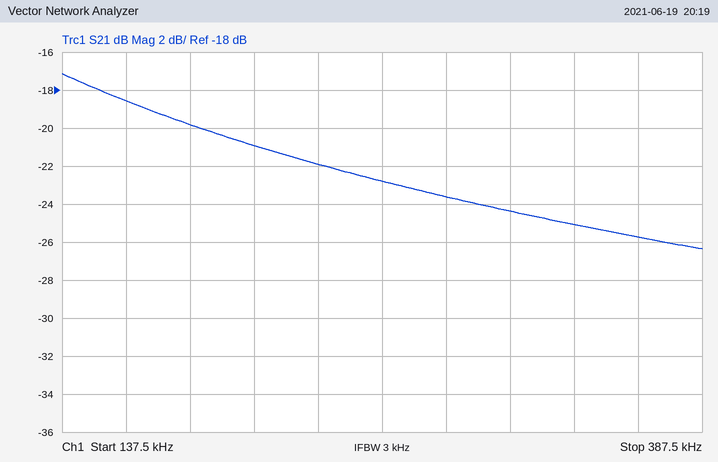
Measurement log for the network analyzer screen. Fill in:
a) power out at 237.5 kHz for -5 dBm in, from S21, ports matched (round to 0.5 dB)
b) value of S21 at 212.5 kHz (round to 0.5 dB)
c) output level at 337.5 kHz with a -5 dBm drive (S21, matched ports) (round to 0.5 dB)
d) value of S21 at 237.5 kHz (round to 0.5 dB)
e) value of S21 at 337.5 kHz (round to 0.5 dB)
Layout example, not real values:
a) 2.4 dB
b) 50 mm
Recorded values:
a) -27.0 dBm
b) -21.0 dB
c) -30.0 dBm
d) -22.0 dB
e) -25.0 dB
